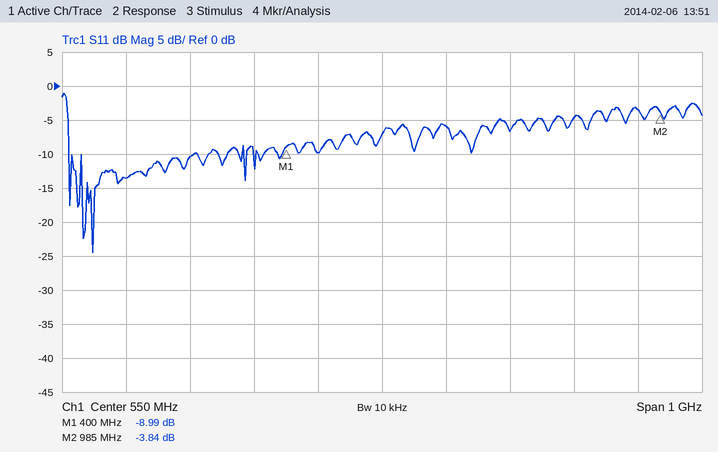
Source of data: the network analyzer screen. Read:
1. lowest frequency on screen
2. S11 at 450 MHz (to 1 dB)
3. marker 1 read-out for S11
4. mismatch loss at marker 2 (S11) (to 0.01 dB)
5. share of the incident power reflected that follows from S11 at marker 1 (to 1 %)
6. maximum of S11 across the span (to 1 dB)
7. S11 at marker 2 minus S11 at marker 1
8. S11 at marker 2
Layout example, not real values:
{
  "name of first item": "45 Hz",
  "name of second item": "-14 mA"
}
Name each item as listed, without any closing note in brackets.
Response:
{
  "lowest frequency on screen": "50 MHz",
  "S11 at 450 MHz": "-10 dB",
  "marker 1 read-out for S11": "-8.99 dB",
  "mismatch loss at marker 2 (S11)": "2.31 dB",
  "share of the incident power reflected that follows from S11 at marker 1": "13 %",
  "maximum of S11 across the span": "-1 dB",
  "S11 at marker 2 minus S11 at marker 1": "5.15 dB",
  "S11 at marker 2": "-3.84 dB"
}
